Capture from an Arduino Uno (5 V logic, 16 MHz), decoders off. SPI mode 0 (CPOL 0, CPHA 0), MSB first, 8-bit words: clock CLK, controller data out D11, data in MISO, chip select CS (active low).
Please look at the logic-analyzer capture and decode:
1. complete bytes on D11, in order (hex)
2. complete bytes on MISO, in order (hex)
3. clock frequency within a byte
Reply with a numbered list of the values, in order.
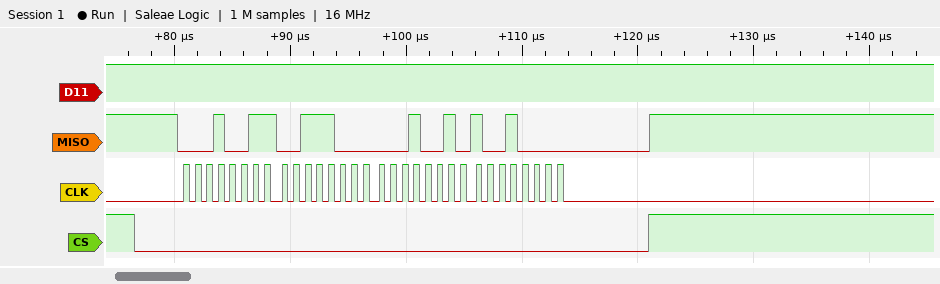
1. FF FF FF FF
2. 13 38 12 90
3. 1 MHz
